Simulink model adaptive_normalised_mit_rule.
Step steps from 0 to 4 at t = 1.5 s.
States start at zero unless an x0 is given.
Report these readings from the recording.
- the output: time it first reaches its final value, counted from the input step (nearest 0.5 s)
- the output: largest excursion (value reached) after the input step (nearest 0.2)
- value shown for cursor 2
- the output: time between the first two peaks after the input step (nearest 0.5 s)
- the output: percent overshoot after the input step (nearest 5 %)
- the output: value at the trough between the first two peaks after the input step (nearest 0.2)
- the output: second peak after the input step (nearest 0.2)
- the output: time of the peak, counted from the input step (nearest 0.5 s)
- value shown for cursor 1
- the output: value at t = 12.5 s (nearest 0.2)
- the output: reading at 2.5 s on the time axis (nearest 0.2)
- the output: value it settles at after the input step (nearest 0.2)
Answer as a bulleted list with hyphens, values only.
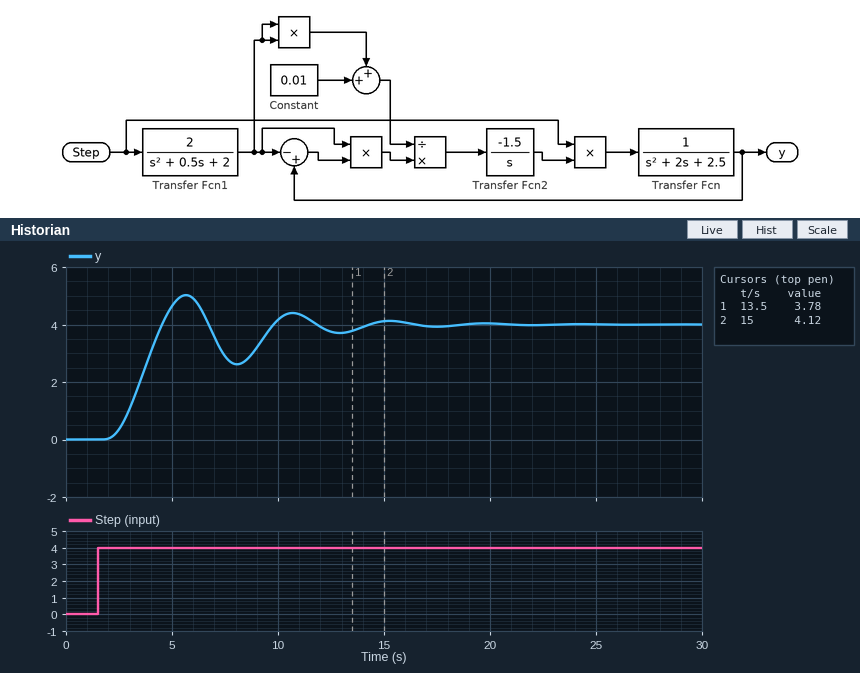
- 3.0 s
- 5.0
- 4.12
- 5.0 s
- 25 %
- 2.6
- 4.4
- 4.0 s
- 3.78
- 3.8
- 0.4
- 4.0
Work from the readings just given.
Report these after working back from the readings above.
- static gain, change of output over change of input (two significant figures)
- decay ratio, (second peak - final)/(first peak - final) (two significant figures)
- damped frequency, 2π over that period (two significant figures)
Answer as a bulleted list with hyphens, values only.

- 1.0
- 0.40
- 1.3 rad/s
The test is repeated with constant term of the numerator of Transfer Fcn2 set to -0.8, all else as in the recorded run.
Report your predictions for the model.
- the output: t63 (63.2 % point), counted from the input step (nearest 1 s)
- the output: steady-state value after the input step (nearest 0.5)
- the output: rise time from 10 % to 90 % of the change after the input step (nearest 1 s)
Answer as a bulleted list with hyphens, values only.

- 3 s
- 4.0
- 7 s
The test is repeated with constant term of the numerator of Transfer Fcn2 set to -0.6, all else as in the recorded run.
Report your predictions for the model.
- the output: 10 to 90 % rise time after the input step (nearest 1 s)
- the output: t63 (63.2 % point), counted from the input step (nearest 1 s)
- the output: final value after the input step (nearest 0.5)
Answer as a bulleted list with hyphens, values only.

- 7 s
- 4 s
- 4.0
